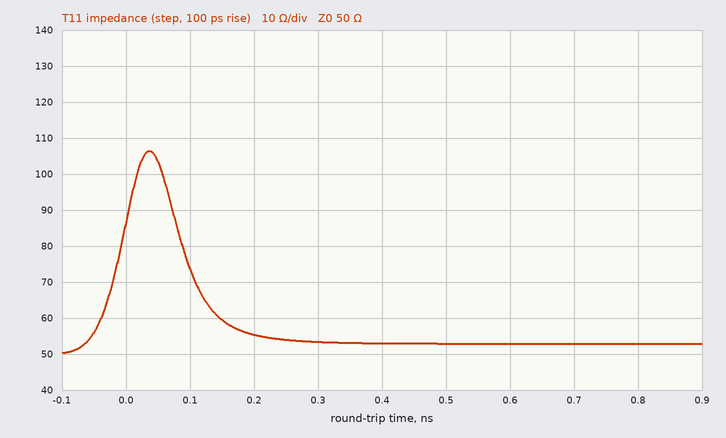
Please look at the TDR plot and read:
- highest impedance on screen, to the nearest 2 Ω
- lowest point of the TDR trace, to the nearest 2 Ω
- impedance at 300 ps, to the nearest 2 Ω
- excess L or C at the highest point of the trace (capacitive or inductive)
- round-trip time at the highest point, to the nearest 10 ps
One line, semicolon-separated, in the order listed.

106 Ω; 50 Ω; 54 Ω; inductive; 40 ps
